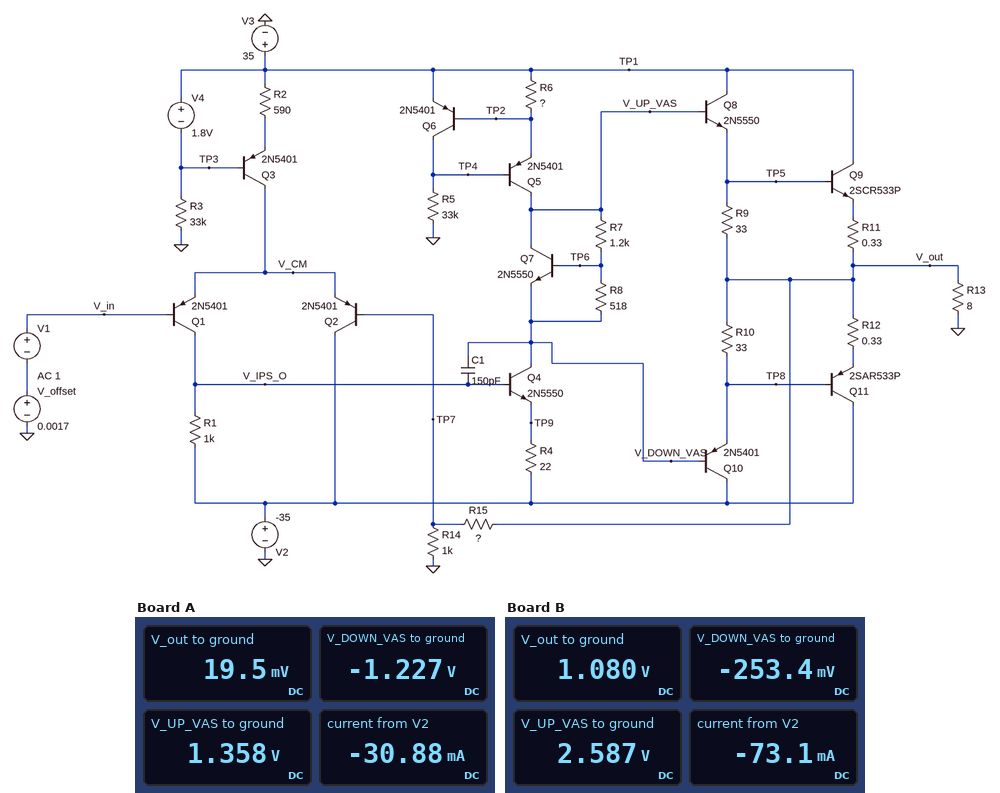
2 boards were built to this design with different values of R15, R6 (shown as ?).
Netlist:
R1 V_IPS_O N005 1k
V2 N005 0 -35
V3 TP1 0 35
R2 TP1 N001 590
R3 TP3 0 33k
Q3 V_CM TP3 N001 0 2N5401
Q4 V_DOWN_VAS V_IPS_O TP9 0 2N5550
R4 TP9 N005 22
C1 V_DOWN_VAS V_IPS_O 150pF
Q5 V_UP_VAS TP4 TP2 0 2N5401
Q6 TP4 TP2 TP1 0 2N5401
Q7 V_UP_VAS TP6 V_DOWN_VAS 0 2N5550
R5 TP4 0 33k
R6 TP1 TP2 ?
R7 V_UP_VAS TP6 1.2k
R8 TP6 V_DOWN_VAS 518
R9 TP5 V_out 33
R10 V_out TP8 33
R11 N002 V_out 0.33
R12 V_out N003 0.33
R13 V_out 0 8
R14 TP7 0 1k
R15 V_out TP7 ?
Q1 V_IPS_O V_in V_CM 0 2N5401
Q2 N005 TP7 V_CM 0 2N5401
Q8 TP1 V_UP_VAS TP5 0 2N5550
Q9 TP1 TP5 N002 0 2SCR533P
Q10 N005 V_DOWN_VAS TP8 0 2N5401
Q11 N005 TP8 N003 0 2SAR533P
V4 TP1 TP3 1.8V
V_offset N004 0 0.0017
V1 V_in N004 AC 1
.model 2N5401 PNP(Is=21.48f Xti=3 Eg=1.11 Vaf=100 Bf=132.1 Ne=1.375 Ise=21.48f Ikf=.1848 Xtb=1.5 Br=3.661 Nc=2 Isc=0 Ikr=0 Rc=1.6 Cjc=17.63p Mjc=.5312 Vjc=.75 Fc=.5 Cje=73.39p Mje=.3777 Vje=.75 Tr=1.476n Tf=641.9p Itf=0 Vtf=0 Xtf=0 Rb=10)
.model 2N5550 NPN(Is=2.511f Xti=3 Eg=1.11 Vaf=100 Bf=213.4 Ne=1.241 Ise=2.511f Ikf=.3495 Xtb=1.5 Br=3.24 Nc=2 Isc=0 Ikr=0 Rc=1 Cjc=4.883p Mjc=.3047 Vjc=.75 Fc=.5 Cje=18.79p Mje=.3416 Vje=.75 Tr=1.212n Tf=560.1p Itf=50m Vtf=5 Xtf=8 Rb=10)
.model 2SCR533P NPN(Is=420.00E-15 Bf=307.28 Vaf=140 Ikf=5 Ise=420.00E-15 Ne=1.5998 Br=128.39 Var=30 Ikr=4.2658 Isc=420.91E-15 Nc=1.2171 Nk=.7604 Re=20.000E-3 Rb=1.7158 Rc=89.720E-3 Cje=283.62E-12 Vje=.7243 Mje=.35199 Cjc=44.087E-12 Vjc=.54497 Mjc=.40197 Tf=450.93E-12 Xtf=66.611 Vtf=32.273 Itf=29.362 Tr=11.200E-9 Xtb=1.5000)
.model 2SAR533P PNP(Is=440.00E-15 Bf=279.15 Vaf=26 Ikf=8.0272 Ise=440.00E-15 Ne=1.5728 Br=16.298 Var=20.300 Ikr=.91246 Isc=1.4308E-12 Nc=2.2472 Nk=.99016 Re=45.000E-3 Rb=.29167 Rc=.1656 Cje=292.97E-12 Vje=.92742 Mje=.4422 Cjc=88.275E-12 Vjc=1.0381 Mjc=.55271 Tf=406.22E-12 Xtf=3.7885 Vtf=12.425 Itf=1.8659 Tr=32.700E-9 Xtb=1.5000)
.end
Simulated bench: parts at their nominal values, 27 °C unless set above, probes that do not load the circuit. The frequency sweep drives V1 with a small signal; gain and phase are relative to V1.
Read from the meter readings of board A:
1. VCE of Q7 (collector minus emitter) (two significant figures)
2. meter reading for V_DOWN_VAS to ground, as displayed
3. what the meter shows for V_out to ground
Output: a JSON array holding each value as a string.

["2.6 V", "-1.227 V", "19.5 mV"]
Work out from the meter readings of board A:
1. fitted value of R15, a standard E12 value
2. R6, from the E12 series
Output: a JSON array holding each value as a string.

["6.8 kΩ", "56 Ω"]
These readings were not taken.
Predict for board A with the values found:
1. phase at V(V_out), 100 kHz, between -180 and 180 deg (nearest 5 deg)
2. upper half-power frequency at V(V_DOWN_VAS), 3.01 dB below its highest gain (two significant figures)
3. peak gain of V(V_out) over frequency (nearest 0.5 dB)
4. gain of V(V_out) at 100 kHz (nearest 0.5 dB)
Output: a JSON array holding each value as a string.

["-5 deg", "1.9 MHz", "18.0 dB", "18.0 dB"]
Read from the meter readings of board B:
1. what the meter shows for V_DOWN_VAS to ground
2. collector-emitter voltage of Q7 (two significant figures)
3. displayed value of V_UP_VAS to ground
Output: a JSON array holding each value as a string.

["-253.4 mV", "2.8 V", "2.587 V"]
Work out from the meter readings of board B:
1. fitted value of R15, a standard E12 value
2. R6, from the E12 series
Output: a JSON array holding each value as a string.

["27 kΩ", "22 Ω"]
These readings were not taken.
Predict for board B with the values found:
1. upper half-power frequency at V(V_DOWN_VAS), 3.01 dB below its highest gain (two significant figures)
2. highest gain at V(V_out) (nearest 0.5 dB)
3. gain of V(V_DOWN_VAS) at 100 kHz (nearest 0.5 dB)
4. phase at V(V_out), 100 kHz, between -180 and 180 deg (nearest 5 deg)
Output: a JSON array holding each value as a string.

["450 kHz", "29.0 dB", "29.0 dB", "-15 deg"]
